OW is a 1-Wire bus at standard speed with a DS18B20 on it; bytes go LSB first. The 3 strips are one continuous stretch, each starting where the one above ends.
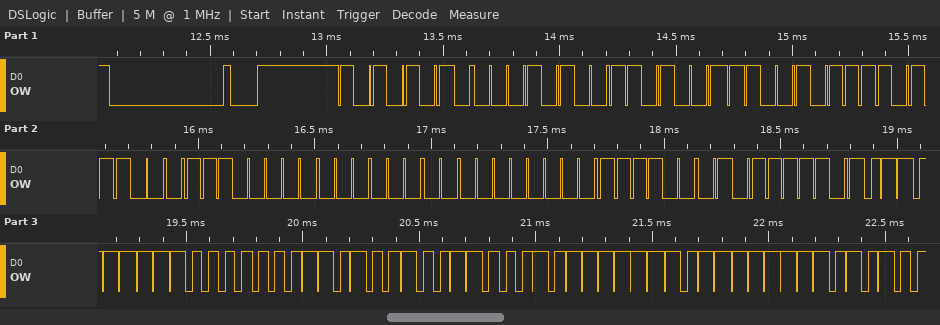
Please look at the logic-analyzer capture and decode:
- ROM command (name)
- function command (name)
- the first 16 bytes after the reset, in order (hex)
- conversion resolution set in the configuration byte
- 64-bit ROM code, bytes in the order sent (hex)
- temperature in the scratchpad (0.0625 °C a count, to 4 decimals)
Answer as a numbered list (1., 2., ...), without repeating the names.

1. Match ROM
2. Read Scratchpad
3. 55 28 CB E9 1D 07 00 00 8F BE F6 01 4B 46 7F FF
4. 12 bits
5. 28 CB E9 1D 07 00 00 8F
6. 31.3750 °C
